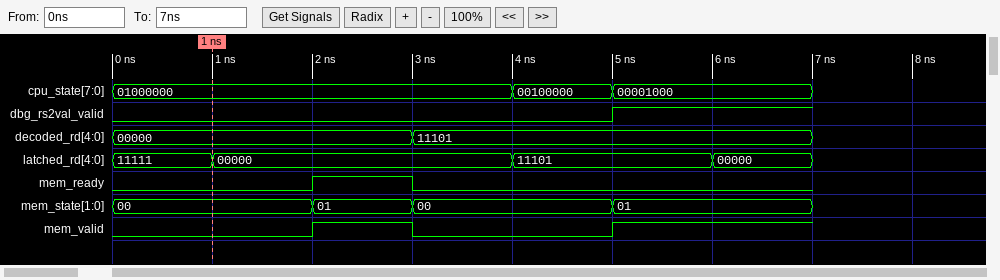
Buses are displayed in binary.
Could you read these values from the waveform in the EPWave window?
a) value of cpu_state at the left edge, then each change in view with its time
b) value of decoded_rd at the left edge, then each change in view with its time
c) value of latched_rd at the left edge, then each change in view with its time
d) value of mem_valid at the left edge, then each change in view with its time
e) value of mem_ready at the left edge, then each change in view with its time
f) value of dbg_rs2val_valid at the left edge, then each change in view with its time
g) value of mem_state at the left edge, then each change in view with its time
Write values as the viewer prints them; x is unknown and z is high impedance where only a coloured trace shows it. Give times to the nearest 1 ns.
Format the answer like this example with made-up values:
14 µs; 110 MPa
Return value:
01000000, 00100000 at 4 ns, 00001000 at 5 ns; 00000, 11101 at 3 ns; 11111, 00000 at 1 ns, 11101 at 4 ns, 00000 at 6 ns; 0, 1 at 2 ns, 0 at 3 ns, 1 at 5 ns; 0, 1 at 2 ns, 0 at 3 ns; 0, 1 at 5 ns; 00, 01 at 2 ns, 00 at 3 ns, 01 at 5 ns
